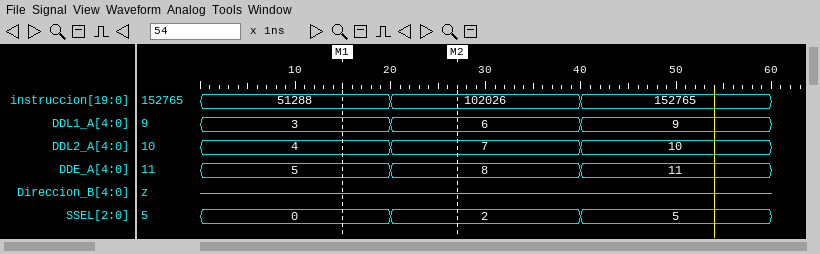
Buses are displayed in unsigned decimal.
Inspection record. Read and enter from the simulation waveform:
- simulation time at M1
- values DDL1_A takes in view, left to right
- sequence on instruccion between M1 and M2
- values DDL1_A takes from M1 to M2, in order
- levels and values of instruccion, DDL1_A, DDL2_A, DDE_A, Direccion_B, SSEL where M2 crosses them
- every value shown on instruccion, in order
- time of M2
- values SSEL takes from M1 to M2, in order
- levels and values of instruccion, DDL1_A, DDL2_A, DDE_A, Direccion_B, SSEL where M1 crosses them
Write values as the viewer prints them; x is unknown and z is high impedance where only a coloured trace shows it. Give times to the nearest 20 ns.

20 ns
3, 6, 9
51288, 102026
3, 6
instruccion=102026, DDL1_A=6, DDL2_A=7, DDE_A=8, Direccion_B=z, SSEL=2
51288, 102026, 152765
20 ns
0, 2
instruccion=51288, DDL1_A=3, DDL2_A=4, DDE_A=5, Direccion_B=z, SSEL=0
